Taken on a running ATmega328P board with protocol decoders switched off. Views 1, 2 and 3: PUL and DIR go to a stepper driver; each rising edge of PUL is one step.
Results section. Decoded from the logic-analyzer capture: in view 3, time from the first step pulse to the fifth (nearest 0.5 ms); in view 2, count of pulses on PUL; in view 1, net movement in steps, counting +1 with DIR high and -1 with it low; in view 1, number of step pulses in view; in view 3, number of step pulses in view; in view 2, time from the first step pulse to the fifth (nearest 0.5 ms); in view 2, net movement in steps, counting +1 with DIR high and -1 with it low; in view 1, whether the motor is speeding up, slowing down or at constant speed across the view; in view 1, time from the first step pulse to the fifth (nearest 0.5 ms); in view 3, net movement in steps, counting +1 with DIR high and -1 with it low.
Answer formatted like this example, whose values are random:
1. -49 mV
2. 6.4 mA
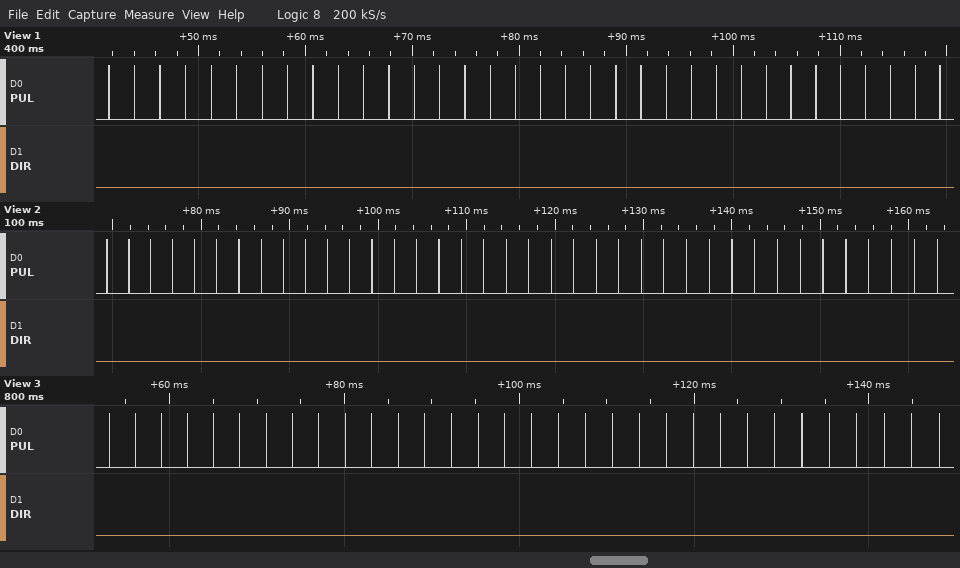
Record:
1. 12.0 ms
2. 38
3. -34
4. 34
5. 32
6. 10.0 ms
7. -38
8. constant speed
9. 9.5 ms
10. -32
